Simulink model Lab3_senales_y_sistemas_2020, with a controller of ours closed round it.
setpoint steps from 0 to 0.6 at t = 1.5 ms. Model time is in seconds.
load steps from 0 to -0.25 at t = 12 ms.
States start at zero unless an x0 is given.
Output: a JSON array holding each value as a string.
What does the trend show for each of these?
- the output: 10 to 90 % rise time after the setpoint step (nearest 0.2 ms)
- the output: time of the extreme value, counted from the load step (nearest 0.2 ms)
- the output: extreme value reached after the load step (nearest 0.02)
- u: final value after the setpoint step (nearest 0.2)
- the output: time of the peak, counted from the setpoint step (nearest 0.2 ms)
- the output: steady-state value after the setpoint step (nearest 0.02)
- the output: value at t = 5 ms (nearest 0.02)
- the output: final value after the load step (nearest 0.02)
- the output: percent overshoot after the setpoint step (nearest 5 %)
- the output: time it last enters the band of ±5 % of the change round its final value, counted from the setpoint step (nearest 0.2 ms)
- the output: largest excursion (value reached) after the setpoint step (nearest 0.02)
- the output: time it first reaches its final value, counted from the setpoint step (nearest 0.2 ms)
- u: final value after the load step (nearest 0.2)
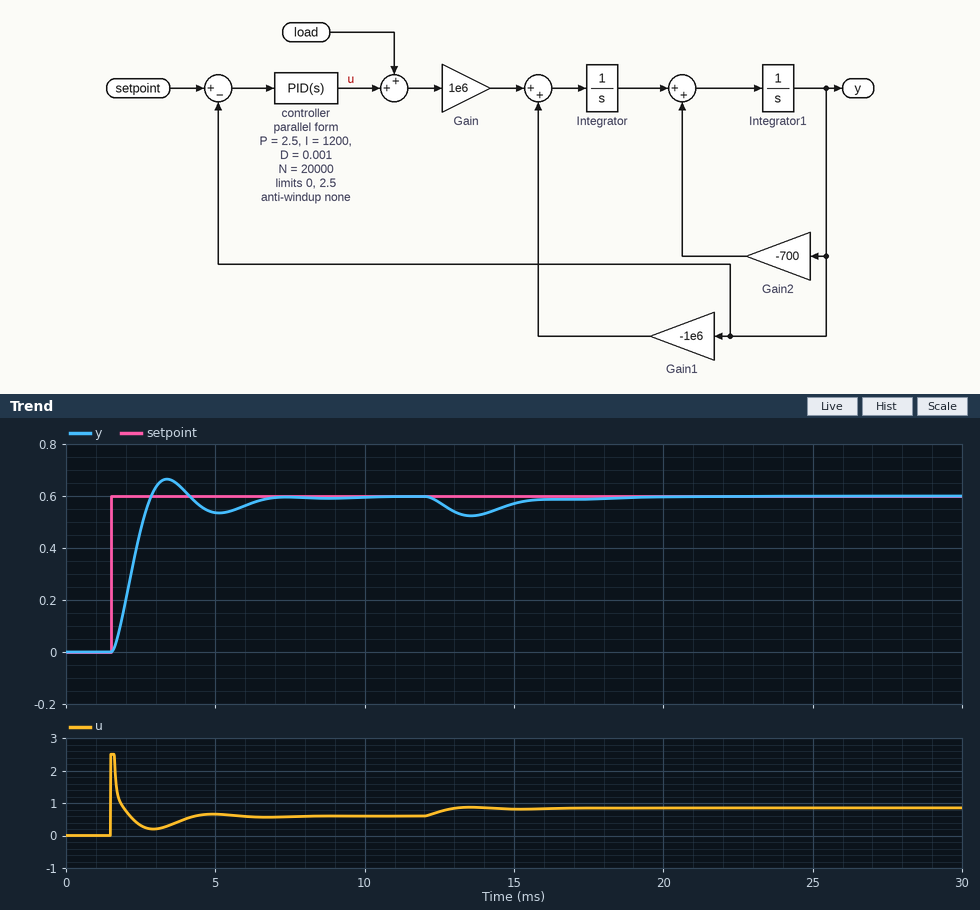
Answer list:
["1.0 ms", "1.6 ms", "0.52", "0.6", "1.8 ms", "0.60", "0.54", "0.60", "10 %", "4.6 ms", "0.66", "1.4 ms", "0.8"]
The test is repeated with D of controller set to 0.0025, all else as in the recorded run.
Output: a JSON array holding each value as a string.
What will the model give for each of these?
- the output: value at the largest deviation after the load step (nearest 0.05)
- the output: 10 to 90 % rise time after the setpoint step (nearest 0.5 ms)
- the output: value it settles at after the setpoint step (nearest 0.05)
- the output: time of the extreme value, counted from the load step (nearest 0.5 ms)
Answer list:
["0.55", "1.5 ms", "0.60", "2.0 ms"]
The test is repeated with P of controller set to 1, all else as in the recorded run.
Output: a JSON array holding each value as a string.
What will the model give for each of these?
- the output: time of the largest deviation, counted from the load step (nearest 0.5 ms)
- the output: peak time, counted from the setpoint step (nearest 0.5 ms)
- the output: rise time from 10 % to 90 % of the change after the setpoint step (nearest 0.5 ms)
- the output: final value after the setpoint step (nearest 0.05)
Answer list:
["2.0 ms", "3.0 ms", "1.5 ms", "0.60"]
